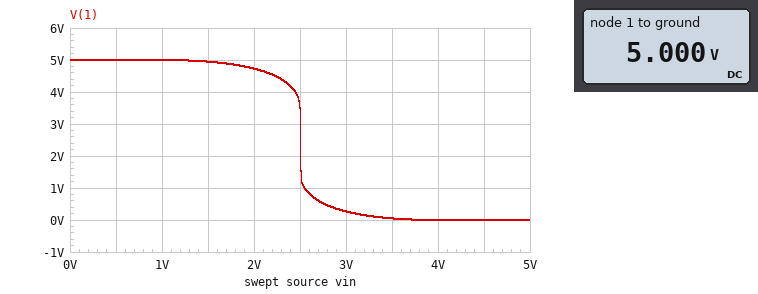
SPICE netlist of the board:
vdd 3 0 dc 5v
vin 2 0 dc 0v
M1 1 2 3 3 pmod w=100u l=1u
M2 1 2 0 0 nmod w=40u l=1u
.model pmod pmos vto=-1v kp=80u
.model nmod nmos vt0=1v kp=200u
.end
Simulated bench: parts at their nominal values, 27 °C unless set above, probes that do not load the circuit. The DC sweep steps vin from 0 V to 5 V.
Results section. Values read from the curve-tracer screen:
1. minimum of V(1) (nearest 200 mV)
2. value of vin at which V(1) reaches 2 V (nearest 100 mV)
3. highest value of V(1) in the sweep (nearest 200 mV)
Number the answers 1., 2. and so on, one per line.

1. 0 V
2. 2.5 V
3. 5.0 V
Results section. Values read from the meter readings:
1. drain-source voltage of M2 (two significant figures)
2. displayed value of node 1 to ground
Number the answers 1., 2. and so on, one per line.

1. 5.0 V
2. 5.000 V
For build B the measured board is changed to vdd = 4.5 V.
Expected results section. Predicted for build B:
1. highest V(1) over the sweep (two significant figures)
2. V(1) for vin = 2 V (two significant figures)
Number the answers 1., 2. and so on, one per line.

1. 4.5 V
2. 4.1 V
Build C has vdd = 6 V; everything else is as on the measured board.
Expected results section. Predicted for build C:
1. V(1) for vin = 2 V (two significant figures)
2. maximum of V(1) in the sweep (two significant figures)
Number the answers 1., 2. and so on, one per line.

1. 5.8 V
2. 6.0 V
